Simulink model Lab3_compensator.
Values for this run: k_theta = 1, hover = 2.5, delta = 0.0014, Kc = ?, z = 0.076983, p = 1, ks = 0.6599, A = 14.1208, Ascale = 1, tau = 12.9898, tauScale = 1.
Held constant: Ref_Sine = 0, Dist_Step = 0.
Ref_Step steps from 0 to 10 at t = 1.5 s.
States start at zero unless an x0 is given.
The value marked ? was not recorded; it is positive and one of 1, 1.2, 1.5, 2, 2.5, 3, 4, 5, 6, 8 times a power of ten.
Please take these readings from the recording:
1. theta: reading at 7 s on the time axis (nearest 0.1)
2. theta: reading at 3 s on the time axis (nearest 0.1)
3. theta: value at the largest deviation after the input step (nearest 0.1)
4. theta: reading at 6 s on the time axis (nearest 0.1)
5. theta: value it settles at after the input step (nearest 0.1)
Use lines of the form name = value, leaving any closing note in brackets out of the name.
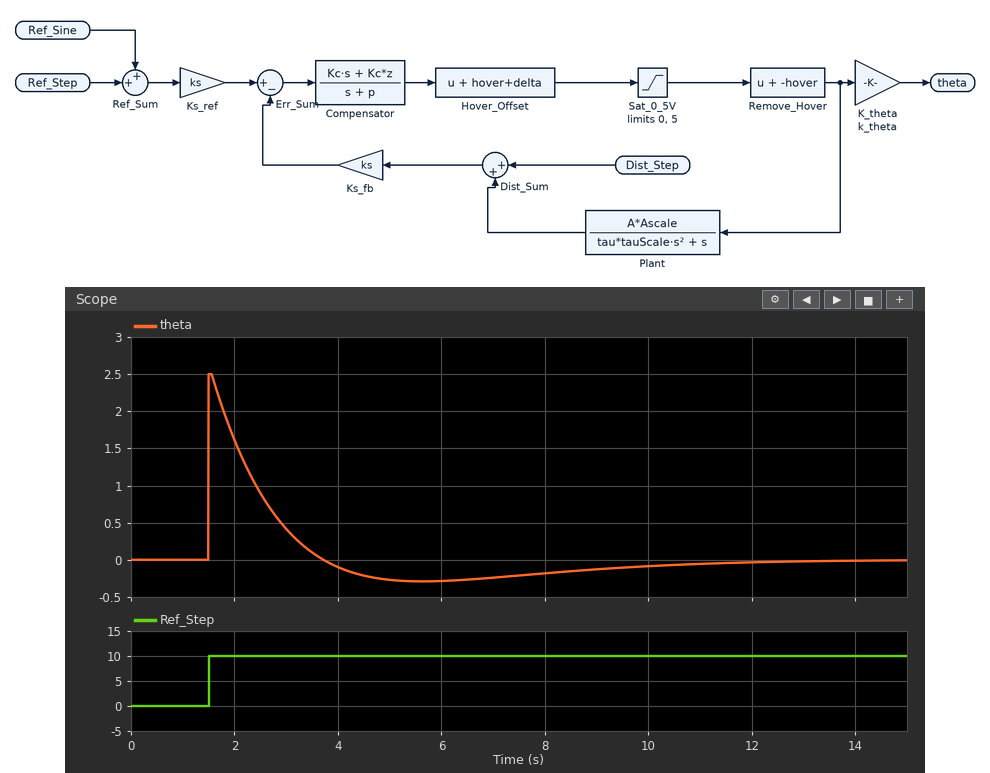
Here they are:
theta: reading at 7 s on the time axis = -0.2
theta: reading at 3 s on the time axis = 0.4
theta: value at the largest deviation after the input step = 2.5
theta: reading at 6 s on the time axis = -0.3
theta: value it settles at after the input step = 0.0
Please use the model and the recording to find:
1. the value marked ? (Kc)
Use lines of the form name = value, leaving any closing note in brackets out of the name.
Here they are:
the value marked ? = 0.4
